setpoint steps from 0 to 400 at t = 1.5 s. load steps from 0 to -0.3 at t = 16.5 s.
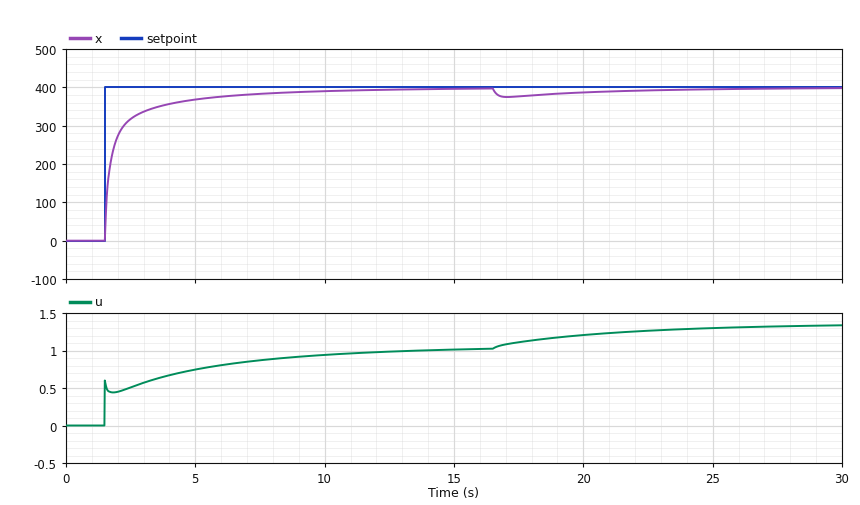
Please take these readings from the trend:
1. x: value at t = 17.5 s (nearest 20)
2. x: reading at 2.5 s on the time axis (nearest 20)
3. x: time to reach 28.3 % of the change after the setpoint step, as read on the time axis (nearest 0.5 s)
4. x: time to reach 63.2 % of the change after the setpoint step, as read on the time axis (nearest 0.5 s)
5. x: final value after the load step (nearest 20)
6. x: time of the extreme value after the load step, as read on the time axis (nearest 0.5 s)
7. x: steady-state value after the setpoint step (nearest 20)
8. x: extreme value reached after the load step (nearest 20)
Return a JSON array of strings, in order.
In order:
["380", "320", "1.5 s", "2.0 s", "400", "17.0 s", "400", "380"]
